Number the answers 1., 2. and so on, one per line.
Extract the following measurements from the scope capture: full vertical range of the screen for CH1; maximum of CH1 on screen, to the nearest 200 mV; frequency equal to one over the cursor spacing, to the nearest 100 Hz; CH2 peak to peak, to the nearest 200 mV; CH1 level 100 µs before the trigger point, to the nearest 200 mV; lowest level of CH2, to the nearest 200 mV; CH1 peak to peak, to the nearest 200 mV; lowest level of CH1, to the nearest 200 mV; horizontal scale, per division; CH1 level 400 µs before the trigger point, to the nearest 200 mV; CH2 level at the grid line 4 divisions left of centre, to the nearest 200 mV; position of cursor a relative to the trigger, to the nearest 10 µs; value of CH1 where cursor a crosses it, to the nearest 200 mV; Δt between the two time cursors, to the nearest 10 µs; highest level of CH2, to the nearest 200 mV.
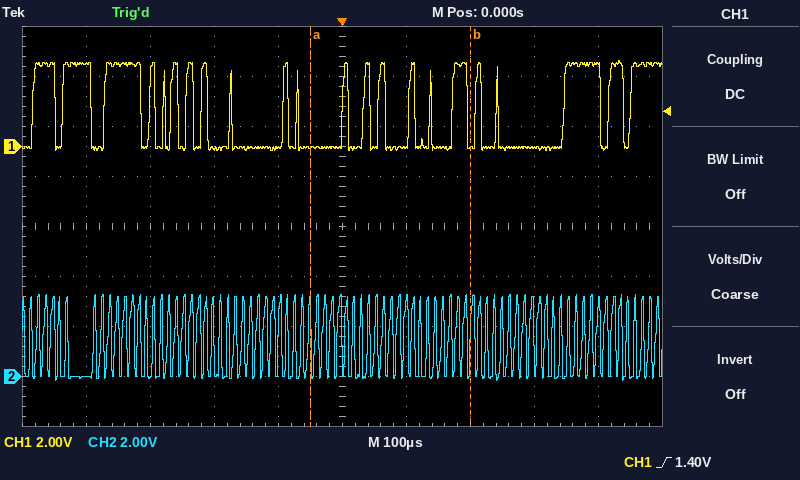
1. 16 V
2. 3.4 V
3. 4.0 kHz
4. 3.4 V
5. 0.0 V
6. -200 mV
7. 3.6 V
8. -200 mV
9. 100 µs
10. 3.4 V
11. 0.0 V
12. -50 µs
13. 0.0 V
14. 250 µs
15. 3.2 V
